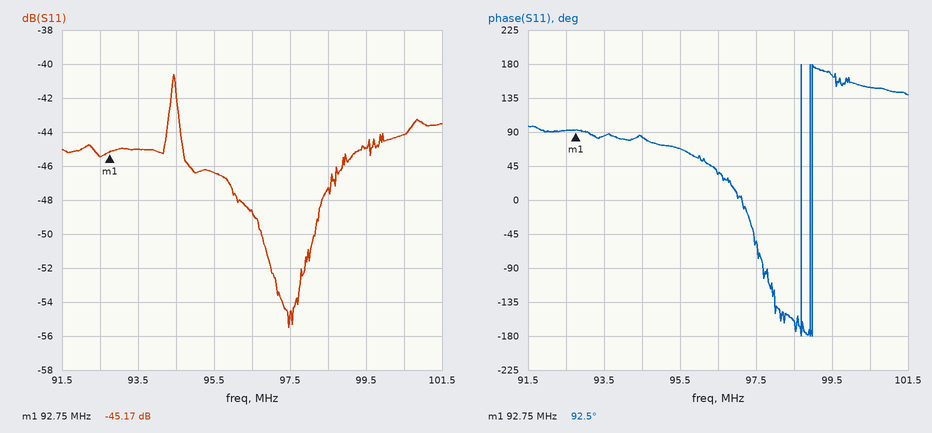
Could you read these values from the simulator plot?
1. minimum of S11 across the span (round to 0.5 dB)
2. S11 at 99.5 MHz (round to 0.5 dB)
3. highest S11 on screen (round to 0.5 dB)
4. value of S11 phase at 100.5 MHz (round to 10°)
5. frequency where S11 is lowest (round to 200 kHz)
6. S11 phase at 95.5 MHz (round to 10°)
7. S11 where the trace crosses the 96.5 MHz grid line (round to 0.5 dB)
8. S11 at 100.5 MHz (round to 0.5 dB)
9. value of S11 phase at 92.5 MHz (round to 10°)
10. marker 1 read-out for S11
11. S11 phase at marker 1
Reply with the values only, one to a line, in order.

-55.5 dB
-45.0 dB
-40.5 dB
150°
97.4 MHz
70°
-48.5 dB
-44.0 dB
90°
-45.17 dB
92.5°
